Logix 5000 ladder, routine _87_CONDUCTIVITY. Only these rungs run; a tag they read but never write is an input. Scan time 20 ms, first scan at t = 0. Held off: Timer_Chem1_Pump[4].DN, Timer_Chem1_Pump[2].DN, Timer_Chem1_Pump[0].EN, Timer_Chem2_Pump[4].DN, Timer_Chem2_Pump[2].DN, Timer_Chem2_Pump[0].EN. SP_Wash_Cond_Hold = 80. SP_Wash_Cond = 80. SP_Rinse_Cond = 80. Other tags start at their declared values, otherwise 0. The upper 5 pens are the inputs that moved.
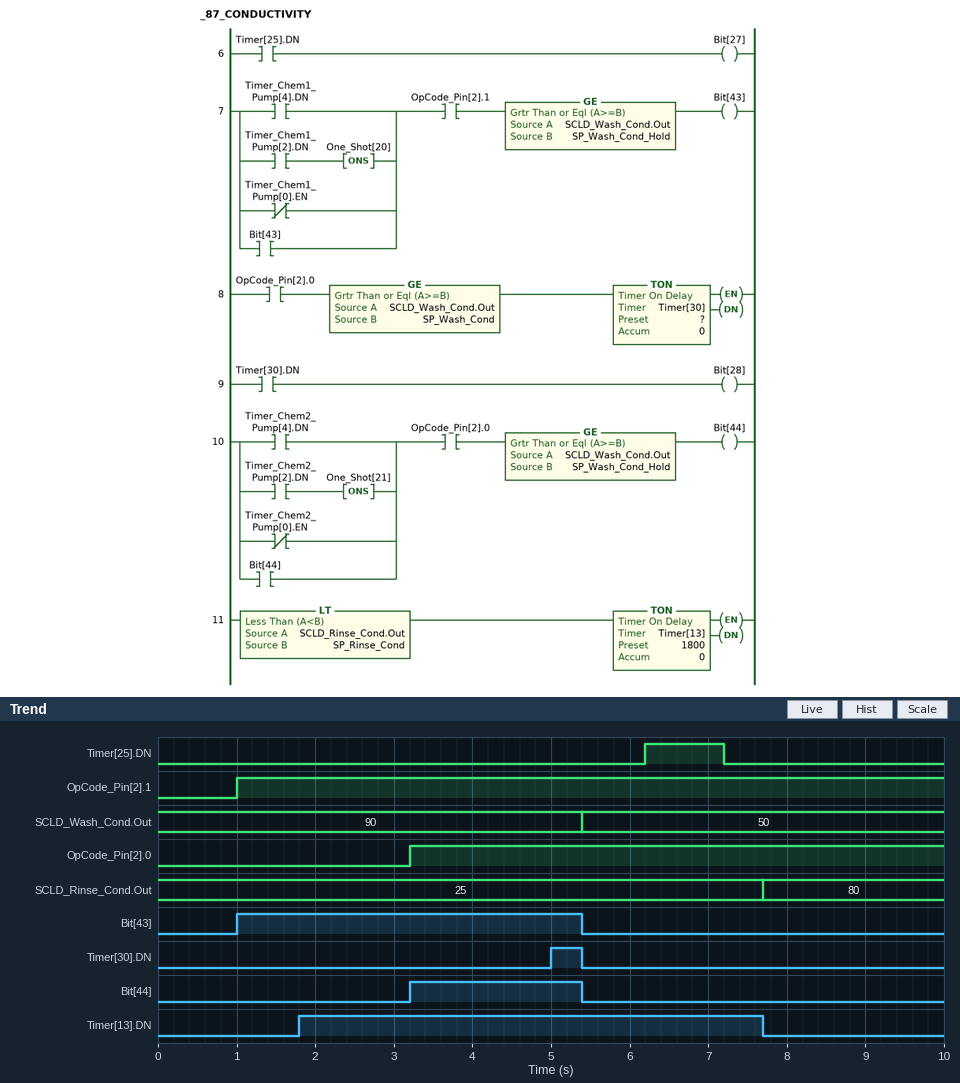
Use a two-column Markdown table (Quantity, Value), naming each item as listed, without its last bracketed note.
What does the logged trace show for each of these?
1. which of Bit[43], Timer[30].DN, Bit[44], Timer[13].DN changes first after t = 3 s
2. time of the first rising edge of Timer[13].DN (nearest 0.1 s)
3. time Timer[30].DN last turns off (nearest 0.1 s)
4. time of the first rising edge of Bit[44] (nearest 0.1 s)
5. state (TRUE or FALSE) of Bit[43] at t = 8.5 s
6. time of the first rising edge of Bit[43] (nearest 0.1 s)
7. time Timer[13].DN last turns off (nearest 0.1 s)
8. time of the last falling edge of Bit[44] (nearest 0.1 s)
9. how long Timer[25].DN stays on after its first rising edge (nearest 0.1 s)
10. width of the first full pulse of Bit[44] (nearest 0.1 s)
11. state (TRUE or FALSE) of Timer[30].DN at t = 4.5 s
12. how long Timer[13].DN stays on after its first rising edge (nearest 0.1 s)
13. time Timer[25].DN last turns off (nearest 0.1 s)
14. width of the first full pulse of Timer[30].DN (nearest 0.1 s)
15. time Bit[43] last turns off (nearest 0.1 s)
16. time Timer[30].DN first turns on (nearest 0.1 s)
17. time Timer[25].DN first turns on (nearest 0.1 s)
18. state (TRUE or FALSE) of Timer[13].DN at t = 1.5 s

| Quantity | Value |
|---|---|
| which of Bit[43], Timer[30].DN, Bit[44], Timer[13].DN changes first after t = 3 s | Bit[44] |
| time of the first rising edge of Timer[13].DN | 1.8 s |
| time Timer[30].DN last turns off | 5.4 s |
| time of the first rising edge of Bit[44] | 3.2 s |
| state (TRUE or FALSE) of Bit[43] at t = 8.5 s | FALSE |
| time of the first rising edge of Bit[43] | 1.0 s |
| time Timer[13].DN last turns off | 7.7 s |
| time of the last falling edge of Bit[44] | 5.4 s |
| how long Timer[25].DN stays on after its first rising edge | 1.0 s |
| width of the first full pulse of Bit[44] | 2.2 s |
| state (TRUE or FALSE) of Timer[30].DN at t = 4.5 s | FALSE |
| how long Timer[13].DN stays on after its first rising edge | 5.9 s |
| time Timer[25].DN last turns off | 7.2 s |
| width of the first full pulse of Timer[30].DN | 0.4 s |
| time Bit[43] last turns off | 5.4 s |
| time Timer[30].DN first turns on | 5.0 s |
| time Timer[25].DN first turns on | 6.2 s |
| state (TRUE or FALSE) of Timer[13].DN at t = 1.5 s | FALSE |
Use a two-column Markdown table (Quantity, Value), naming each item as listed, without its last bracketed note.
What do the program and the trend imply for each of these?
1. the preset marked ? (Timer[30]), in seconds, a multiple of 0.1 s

| Quantity | Value |
|---|---|
| the preset marked ? (Timer[30]), in seconds, a multiple of 0.1 s | 1.8 s |
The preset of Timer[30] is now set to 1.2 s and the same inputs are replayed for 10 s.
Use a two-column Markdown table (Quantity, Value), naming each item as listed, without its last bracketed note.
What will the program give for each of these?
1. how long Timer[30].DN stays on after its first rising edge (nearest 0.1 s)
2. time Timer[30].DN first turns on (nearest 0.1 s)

| Quantity | Value |
|---|---|
| how long Timer[30].DN stays on after its first rising edge | 1.0 s |
| time Timer[30].DN first turns on | 4.4 s |
